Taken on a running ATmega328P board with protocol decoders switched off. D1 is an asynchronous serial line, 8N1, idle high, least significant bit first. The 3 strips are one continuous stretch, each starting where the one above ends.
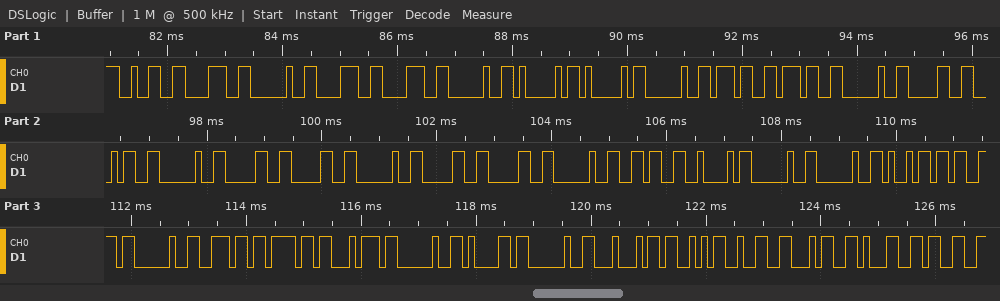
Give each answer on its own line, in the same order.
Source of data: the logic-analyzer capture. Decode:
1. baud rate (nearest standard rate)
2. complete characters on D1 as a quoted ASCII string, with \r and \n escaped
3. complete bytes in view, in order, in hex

9600 baud
"28 88 AA 77 04 00 00 6B  is not a DS2413"
32 38 20 38 38 20 41 41 20 37 37 20 30 34 20 30 30 20 30 30 20 36 42 20 20 69 73 20 6E 6F 74 20 61 20 44 53 32 34 31 33
